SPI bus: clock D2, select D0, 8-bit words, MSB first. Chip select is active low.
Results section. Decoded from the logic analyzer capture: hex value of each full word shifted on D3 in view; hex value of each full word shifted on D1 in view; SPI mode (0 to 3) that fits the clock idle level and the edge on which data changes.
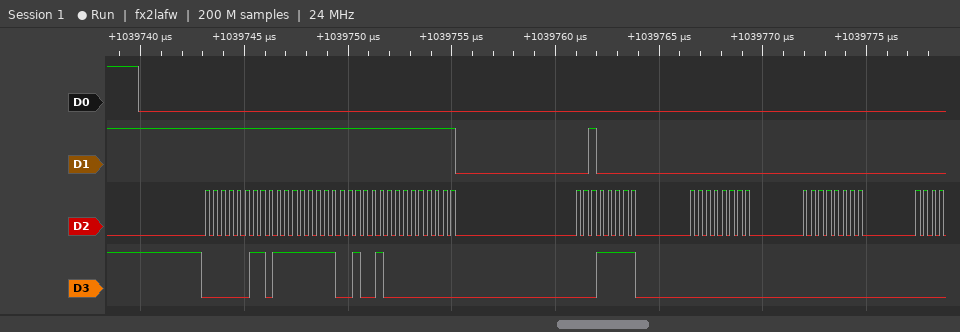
03, 7F, 92, 00, 1F, 00, 00
FF, FF, FF, FF, 20, 00, 00
0
